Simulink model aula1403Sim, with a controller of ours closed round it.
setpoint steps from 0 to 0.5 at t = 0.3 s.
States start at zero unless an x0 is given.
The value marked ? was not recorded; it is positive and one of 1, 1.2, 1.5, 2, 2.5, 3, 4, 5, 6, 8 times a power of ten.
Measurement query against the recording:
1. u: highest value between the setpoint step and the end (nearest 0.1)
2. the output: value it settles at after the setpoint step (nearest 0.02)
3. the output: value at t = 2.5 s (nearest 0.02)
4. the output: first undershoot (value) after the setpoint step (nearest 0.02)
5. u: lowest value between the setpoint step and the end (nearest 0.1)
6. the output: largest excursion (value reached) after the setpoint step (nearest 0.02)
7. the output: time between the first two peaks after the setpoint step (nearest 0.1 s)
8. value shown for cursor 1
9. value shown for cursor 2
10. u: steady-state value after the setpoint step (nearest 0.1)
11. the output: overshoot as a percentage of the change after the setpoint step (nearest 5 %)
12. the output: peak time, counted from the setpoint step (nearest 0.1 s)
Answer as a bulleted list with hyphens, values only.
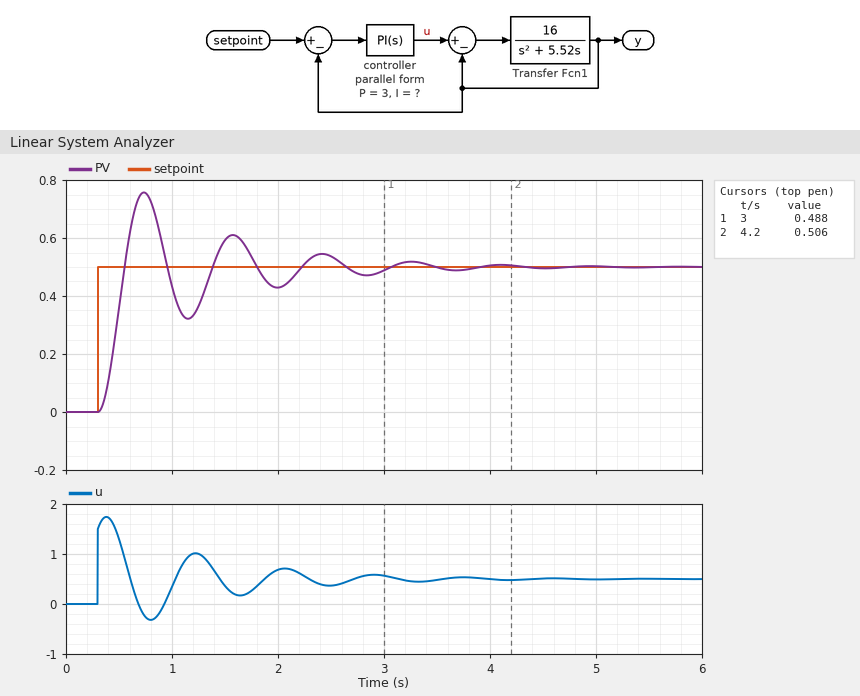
- 1.7
- 0.50
- 0.54
- 0.32
- -0.3
- 0.76
- 0.8 s
- 0.488
- 0.506
- 0.5
- 50 %
- 0.4 s
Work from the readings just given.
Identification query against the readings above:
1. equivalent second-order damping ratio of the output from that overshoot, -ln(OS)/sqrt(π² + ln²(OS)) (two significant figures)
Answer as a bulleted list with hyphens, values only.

- 0.22
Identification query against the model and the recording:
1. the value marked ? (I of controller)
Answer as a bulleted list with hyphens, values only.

- 12
